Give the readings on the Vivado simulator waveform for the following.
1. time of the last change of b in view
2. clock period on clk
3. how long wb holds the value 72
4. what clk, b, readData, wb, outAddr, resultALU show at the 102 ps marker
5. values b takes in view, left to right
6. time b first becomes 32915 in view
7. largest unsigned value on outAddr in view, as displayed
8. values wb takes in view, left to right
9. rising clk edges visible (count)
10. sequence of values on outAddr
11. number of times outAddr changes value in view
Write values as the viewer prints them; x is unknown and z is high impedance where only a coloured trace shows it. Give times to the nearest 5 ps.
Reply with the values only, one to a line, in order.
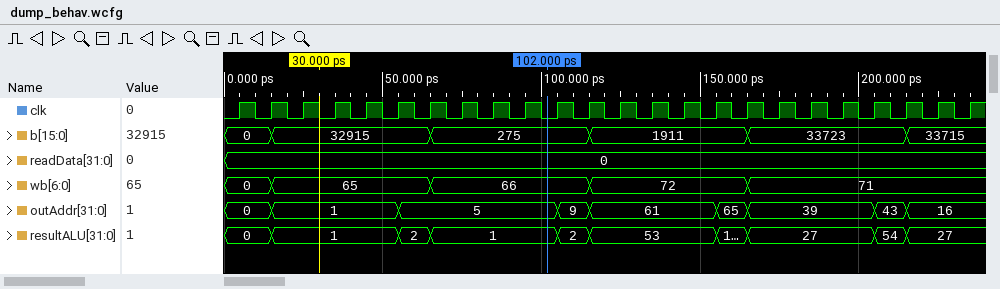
215 ps
10 ps
50 ps
clk=0, b=275, readData=0, wb=66, outAddr=5, resultALU=1
0, 32915, 275, 1911, 33723, 33715
15 ps
65
0, 65, 66, 72, 71
24
0, 1, 5, 9, 61, 65, 39, 43, 16
8
